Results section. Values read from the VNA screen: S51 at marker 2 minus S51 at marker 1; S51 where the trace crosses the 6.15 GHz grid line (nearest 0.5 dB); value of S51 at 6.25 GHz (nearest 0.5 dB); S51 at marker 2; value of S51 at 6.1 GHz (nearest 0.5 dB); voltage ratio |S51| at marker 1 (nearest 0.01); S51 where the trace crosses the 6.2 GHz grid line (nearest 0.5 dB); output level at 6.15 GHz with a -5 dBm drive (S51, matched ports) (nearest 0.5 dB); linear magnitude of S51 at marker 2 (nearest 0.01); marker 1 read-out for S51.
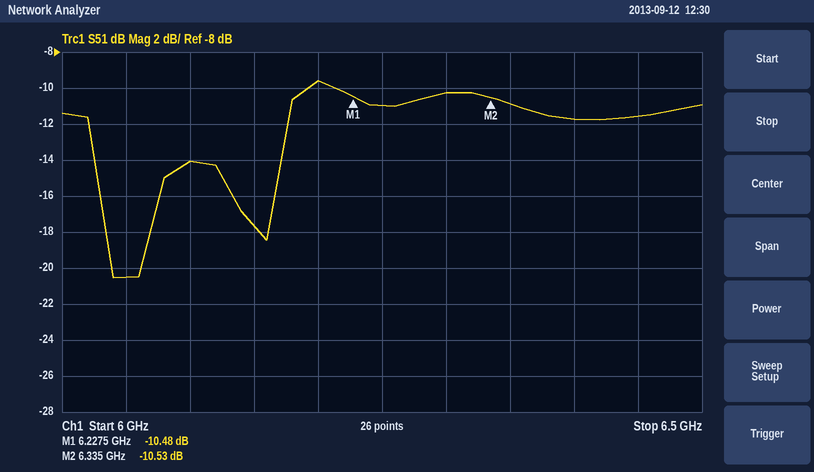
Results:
-0.05 dB
-17.5 dB
-11.0 dB
-10.53 dB
-14.0 dB
0.30
-9.5 dB
-22.5 dBm
0.30
-10.48 dB
